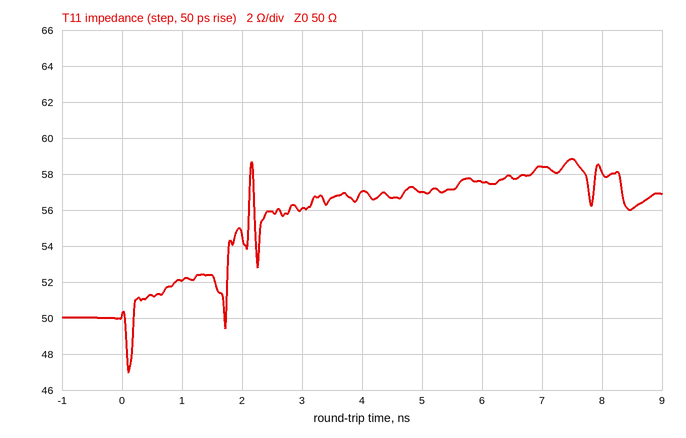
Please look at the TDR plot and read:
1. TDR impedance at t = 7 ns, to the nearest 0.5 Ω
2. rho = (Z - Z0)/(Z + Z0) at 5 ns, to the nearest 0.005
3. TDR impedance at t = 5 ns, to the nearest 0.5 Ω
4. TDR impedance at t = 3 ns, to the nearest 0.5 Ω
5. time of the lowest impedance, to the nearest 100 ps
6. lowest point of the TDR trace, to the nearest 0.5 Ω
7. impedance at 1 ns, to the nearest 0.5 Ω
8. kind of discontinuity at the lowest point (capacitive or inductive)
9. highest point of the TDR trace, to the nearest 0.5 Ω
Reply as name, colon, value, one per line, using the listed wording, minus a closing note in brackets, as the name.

TDR impedance at t = 7 ns, to the nearest 0.5 Ω: 58.5 Ω
rho = (Z - Z0)/(Z + Z0) at 5 ns, to the nearest 0.005: +0.065
TDR impedance at t = 5 ns, to the nearest 0.5 Ω: 57.0 Ω
TDR impedance at t = 3 ns, to the nearest 0.5 Ω: 56.0 Ω
time of the lowest impedance, to the nearest 100 ps: 100 ps
lowest point of the TDR trace, to the nearest 0.5 Ω: 47.0 Ω
impedance at 1 ns, to the nearest 0.5 Ω: 52.0 Ω
kind of discontinuity at the lowest point: capacitive
highest point of the TDR trace, to the nearest 0.5 Ω: 59.0 Ω
